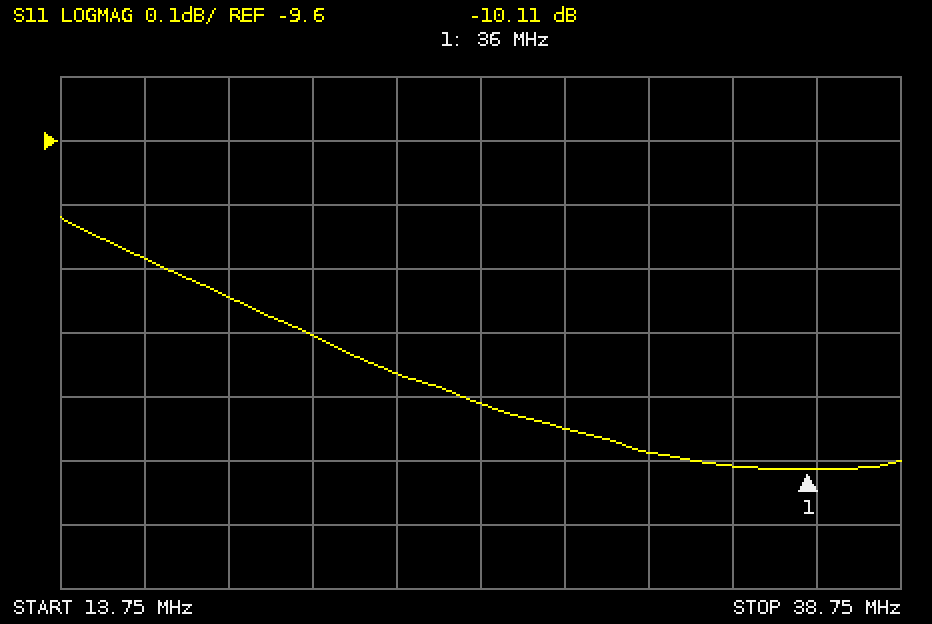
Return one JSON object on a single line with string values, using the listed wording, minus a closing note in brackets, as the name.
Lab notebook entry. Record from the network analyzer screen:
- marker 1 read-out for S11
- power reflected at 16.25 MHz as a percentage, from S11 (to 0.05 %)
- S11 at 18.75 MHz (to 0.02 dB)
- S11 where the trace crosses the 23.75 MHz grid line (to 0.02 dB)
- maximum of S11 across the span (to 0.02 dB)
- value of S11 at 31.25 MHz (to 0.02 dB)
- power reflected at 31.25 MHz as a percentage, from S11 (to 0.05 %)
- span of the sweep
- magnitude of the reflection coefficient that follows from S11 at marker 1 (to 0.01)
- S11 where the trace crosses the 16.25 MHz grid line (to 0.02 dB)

{"marker 1 read-out for S11": "-10.11 dB", "power reflected at 16.25 MHz as a percentage, from S11": "10.50 %", "S11 at 18.75 MHz": "-9.84 dB", "S11 where the trace crosses the 23.75 MHz grid line": "-9.96 dB", "maximum of S11 across the span": "-9.72 dB", "value of S11 at 31.25 MHz": "-10.08 dB", "power reflected at 31.25 MHz as a percentage, from S11": "9.80 %", "span of the sweep": "25 MHz", "magnitude of the reflection coefficient that follows from S11 at marker 1": "0.31", "S11 where the trace crosses the 16.25 MHz grid line": "-9.78 dB"}
